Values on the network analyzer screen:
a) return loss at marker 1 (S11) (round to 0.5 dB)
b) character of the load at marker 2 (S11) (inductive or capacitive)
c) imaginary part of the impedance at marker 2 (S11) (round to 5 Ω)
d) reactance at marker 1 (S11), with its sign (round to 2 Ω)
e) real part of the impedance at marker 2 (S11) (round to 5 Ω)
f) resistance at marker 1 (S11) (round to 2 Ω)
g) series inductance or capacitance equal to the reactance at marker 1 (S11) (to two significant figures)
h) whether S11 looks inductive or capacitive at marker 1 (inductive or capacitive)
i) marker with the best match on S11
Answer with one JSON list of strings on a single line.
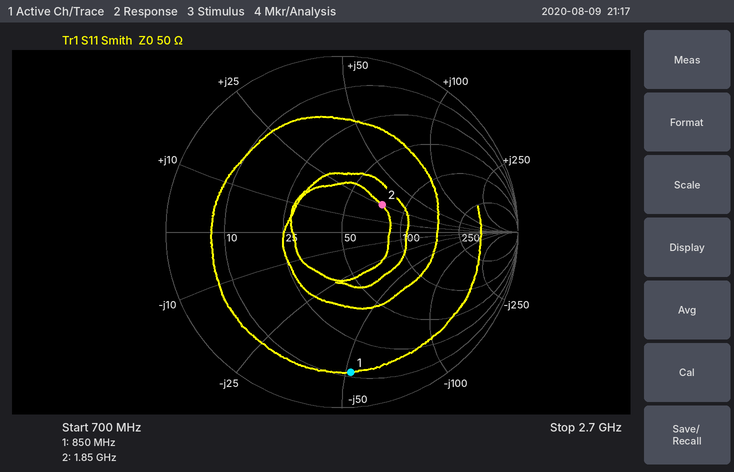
["2.0 dB", "inductive", "+25 Ω", "-52 Ω", "75 Ω", "12 Ω", "3.6 pF", "capacitive", "marker 2"]
